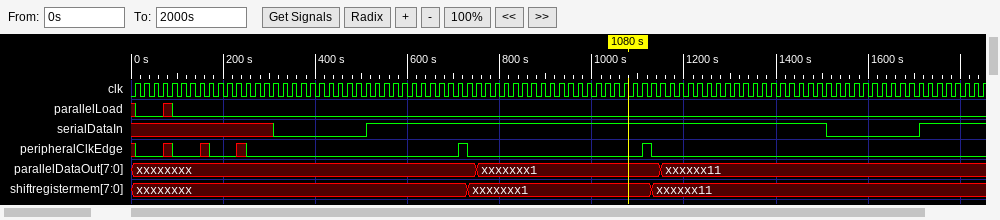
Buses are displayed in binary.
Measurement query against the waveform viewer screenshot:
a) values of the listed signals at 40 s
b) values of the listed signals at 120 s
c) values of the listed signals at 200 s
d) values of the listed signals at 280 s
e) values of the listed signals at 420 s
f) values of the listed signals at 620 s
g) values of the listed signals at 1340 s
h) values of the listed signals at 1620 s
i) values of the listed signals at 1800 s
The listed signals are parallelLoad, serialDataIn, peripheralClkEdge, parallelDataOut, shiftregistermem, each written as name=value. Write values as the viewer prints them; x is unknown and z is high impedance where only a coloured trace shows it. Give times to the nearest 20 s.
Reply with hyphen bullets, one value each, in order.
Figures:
- parallelLoad=0, serialDataIn=x, peripheralClkEdge=0, parallelDataOut=xxxxxxxx, shiftregistermem=xxxxxxxx
- parallelLoad=0, serialDataIn=x, peripheralClkEdge=0, parallelDataOut=xxxxxxxx, shiftregistermem=xxxxxxxx
- parallelLoad=0, serialDataIn=x, peripheralClkEdge=0, parallelDataOut=xxxxxxxx, shiftregistermem=xxxxxxxx
- parallelLoad=0, serialDataIn=x, peripheralClkEdge=0, parallelDataOut=xxxxxxxx, shiftregistermem=xxxxxxxx
- parallelLoad=0, serialDataIn=0, peripheralClkEdge=0, parallelDataOut=xxxxxxxx, shiftregistermem=xxxxxxxx
- parallelLoad=0, serialDataIn=1, peripheralClkEdge=0, parallelDataOut=xxxxxxxx, shiftregistermem=xxxxxxxx
- parallelLoad=0, serialDataIn=1, peripheralClkEdge=0, parallelDataOut=xxxxxx11, shiftregistermem=xxxxxx11
- parallelLoad=0, serialDataIn=0, peripheralClkEdge=0, parallelDataOut=xxxxxx11, shiftregistermem=xxxxxx11
- parallelLoad=0, serialDataIn=1, peripheralClkEdge=0, parallelDataOut=xxxxxx11, shiftregistermem=xxxxxx11
